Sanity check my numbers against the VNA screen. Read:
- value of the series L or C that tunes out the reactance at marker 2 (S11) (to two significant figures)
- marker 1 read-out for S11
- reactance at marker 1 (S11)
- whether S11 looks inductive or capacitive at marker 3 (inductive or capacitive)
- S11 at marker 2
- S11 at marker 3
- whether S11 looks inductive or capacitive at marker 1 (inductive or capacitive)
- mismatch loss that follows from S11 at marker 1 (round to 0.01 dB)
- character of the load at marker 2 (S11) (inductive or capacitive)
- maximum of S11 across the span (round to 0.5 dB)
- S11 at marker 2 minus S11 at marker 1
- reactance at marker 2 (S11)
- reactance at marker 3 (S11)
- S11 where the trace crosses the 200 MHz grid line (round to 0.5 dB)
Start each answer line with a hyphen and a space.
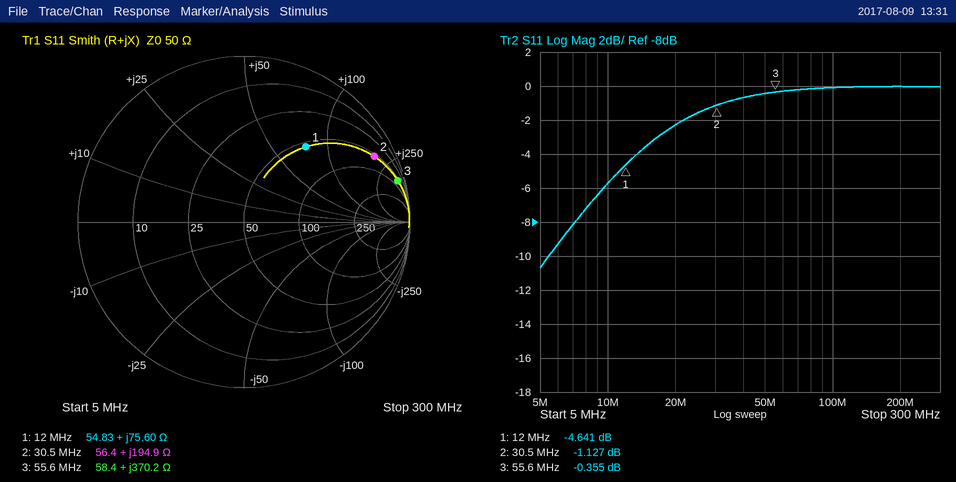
- 27 pF
- -4.641 dB
- +75.60 Ω
- inductive
- -1.127 dB
- -0.355 dB
- inductive
- 1.83 dB
- inductive
- 0.0 dB
- 3.514 dB
- +194.9 Ω
- +370.2 Ω
- 0.0 dB
